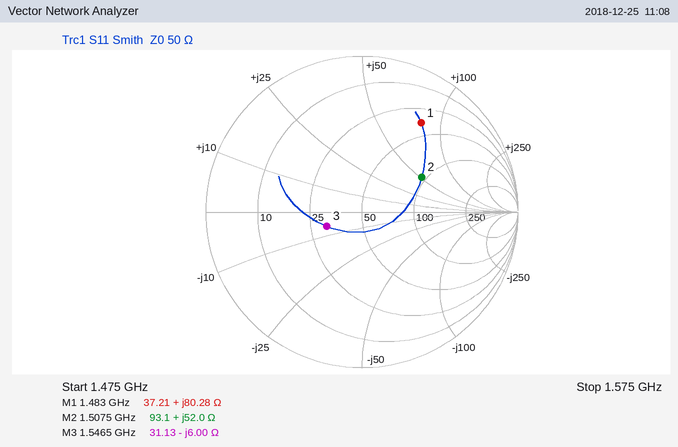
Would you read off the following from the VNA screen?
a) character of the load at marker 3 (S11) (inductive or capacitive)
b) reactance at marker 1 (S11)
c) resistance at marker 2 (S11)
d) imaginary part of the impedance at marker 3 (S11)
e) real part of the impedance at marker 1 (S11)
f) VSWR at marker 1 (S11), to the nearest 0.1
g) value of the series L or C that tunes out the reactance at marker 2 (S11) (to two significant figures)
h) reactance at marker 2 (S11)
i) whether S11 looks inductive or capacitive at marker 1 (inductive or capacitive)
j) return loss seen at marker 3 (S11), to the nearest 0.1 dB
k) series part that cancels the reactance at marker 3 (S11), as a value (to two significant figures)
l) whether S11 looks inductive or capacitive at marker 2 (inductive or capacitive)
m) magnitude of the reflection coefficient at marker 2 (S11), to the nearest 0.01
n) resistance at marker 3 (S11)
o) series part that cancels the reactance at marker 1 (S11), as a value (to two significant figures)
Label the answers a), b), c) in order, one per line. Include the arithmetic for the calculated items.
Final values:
a) capacitive
b) +80.28 Ω
c) 93.1 Ω
d) -6.00 Ω
e) 37.21 Ω
f) 5.4
g) C = 1/(2π × 1.5075 GHz × 52 Ω) ≈ 2.0 pF
h) +52.0 Ω
i) inductive
j) 12.3 dB
k) L = 6 Ω/(2π × 1.5465 GHz) ≈ 617 pH, so 620 pH to two significant figures
l) inductive
m) 0.44
n) 31.13 Ω
o) C = 1/(2π × 1.483 GHz × 80.28 Ω) ≈ 1.3 pF
